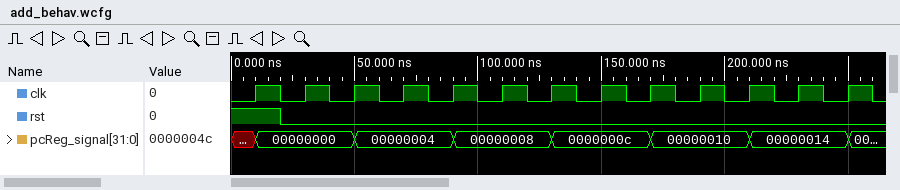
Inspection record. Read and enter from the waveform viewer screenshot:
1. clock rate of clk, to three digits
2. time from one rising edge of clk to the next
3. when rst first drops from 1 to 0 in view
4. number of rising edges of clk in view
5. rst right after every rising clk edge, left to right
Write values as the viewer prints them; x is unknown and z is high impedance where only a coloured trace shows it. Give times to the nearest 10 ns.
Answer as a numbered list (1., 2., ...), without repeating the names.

1. 50.0 MHz
2. 20 ns
3. 20 ns
4. 13
5. 1 0 0 0 0 0 0 0 0 0 0 0 0
